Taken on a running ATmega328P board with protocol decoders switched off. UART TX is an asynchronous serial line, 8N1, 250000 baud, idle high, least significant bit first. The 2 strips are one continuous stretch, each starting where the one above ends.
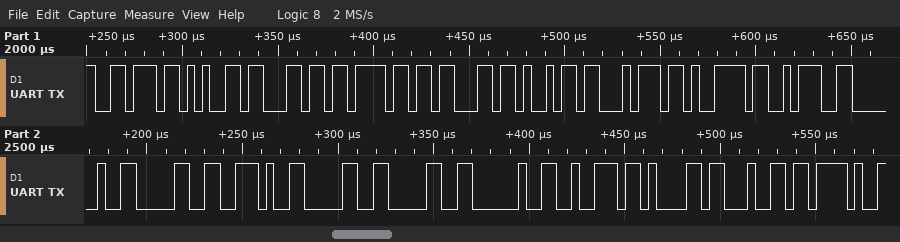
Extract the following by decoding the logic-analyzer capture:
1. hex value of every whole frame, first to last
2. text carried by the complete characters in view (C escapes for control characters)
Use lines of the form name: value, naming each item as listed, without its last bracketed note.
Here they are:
hex value of every whole frame, first to last: 76 65 6C 6F 63 69 74 79 3A 20 30 2E 30 30 20 72 61 64 2F
text carried by the complete characters in view: "velocity: 0.00 rad/"
